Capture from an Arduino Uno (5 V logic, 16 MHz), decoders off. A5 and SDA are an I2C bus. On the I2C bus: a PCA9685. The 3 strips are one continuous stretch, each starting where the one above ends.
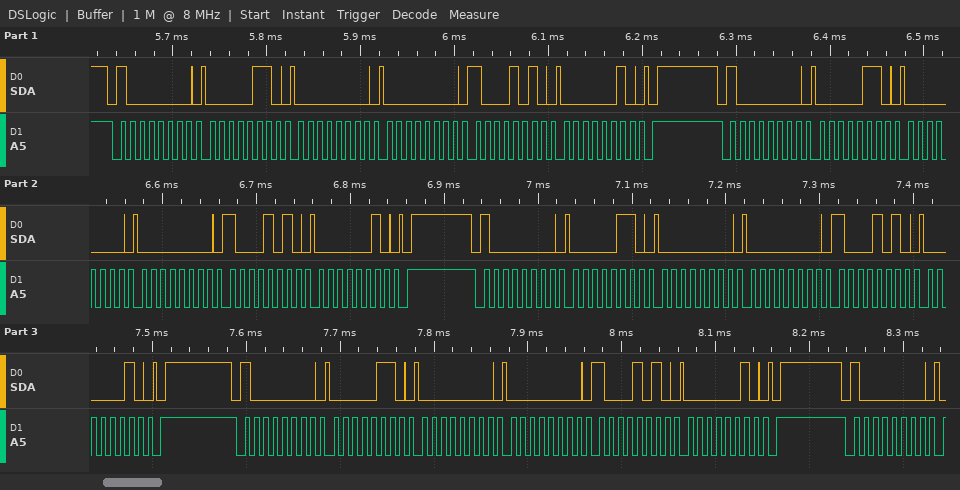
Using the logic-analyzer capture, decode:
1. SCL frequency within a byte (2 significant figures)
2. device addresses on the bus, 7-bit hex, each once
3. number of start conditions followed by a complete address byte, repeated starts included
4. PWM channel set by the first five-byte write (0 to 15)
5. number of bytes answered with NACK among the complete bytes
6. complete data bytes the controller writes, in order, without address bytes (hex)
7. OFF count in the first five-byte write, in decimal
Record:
100 kHz
0x40
5
0
0
06 00 00 8A 02 06 00 00 8A 02 06 00 00 8A 02 06 00 00 8A 02
650
